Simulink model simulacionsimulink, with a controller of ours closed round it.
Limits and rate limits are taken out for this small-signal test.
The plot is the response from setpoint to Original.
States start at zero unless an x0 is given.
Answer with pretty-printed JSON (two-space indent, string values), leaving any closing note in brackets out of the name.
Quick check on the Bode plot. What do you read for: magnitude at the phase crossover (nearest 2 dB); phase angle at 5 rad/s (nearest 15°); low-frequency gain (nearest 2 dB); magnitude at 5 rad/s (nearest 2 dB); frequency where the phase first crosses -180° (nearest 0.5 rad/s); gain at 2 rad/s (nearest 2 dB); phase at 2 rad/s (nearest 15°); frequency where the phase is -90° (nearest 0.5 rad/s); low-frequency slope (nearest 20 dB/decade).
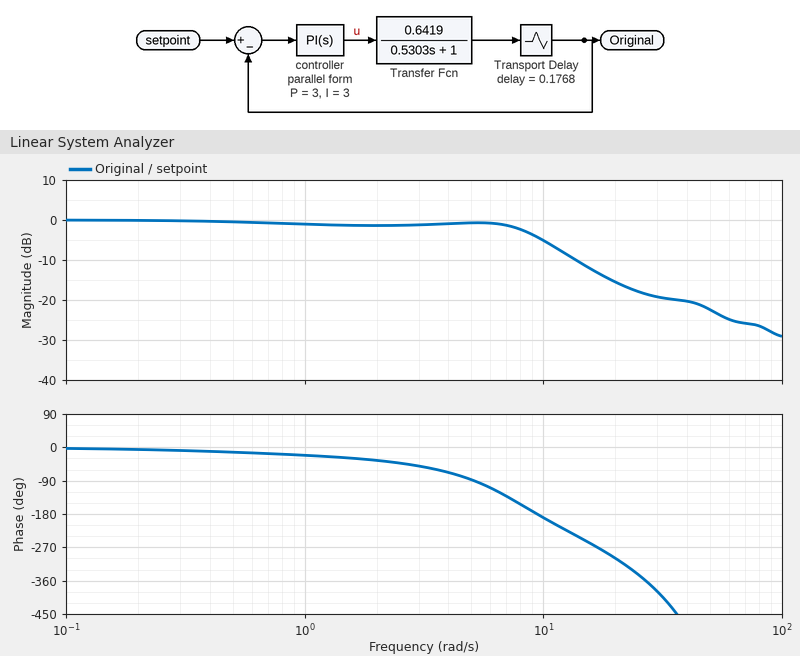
{
  "magnitude at the phase crossover": "-4 dB",
  "phase angle at 5 rad/s": "-90°",
  "low-frequency gain": "0 dB",
  "magnitude at 5 rad/s": "0 dB",
  "frequency where the phase first crosses -180°": "9.5 rad/s",
  "gain at 2 rad/s": "-2 dB",
  "phase at 2 rad/s": "-30°",
  "frequency where the phase is -90°": "5.0 rad/s",
  "low-frequency slope": "0 dB/decade"
}
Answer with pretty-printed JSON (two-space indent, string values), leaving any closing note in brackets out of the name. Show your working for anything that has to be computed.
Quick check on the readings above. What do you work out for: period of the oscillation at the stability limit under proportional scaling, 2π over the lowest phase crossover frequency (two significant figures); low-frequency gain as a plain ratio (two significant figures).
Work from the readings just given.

{
  "period of the oscillation at the stability limit under proportional scaling, 2π over the lowest phase crossover frequency": "2π / 9.5 = 0.66 s",
  "low-frequency gain as a plain ratio": "10^(0 / 20) = 1.0"
}
